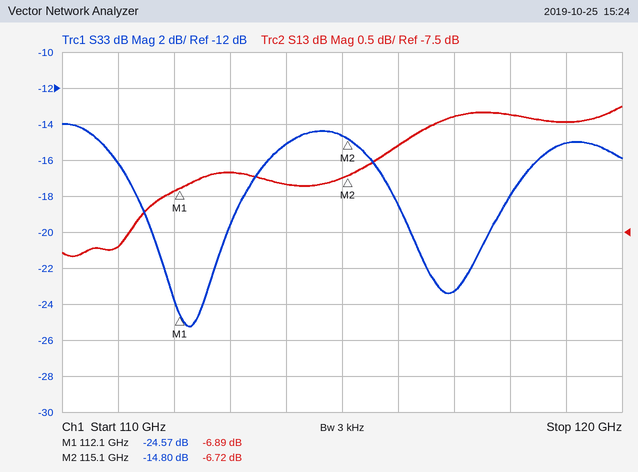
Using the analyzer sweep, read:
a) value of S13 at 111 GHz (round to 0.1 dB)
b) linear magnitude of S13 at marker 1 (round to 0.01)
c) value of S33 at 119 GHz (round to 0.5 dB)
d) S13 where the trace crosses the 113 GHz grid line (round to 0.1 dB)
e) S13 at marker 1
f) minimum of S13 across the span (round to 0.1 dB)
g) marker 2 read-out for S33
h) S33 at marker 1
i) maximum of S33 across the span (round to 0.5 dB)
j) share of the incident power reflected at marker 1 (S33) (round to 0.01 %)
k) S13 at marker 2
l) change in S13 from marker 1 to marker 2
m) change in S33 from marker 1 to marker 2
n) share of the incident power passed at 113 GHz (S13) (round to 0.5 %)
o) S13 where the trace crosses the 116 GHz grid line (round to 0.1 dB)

-7.7 dB
0.45
-15.0 dB
-6.7 dB
-6.89 dB
-7.8 dB
-14.80 dB
-24.57 dB
-14.0 dB
0.35 %
-6.72 dB
0.17 dB
9.77 dB
21.5 %
-6.3 dB
